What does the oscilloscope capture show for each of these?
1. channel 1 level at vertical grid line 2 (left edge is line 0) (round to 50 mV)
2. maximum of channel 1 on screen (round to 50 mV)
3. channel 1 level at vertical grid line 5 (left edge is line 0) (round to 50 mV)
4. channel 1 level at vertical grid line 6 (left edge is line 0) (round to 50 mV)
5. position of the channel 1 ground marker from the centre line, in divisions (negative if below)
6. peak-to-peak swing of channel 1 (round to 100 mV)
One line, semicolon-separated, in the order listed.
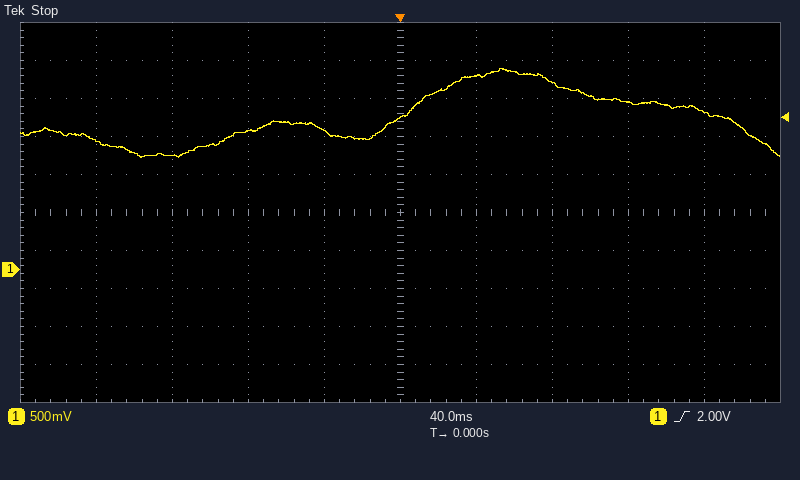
1.50 V; 2.65 V; 2.00 V; 2.55 V; -1.5 div; 1.20 V
